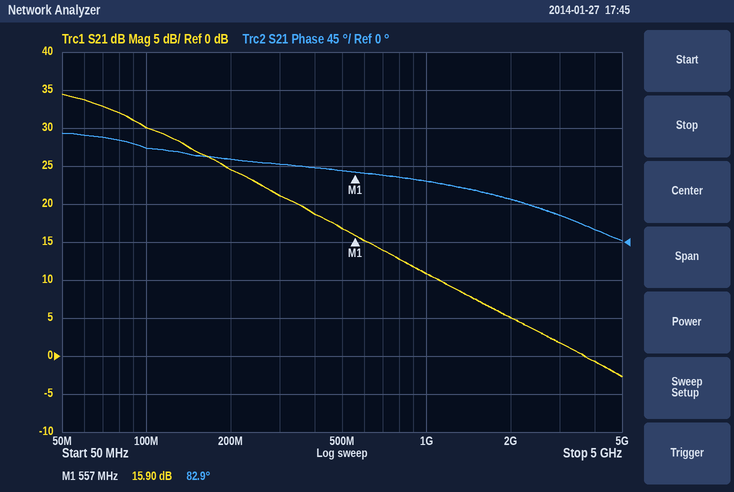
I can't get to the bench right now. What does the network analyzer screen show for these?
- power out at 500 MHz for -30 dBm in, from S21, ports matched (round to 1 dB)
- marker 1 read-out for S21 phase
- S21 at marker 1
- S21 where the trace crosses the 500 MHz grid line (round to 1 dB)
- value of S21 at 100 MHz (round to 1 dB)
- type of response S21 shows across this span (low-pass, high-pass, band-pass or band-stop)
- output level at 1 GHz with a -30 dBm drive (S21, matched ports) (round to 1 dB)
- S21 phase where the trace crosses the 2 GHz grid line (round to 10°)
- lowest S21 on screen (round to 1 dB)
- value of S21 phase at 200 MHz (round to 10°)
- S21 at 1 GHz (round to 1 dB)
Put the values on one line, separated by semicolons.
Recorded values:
-13 dBm; 82.9°; 15.90 dB; 17 dB; 30 dB; low-pass; -19 dBm; 50°; -3 dB; 100°; 11 dB
